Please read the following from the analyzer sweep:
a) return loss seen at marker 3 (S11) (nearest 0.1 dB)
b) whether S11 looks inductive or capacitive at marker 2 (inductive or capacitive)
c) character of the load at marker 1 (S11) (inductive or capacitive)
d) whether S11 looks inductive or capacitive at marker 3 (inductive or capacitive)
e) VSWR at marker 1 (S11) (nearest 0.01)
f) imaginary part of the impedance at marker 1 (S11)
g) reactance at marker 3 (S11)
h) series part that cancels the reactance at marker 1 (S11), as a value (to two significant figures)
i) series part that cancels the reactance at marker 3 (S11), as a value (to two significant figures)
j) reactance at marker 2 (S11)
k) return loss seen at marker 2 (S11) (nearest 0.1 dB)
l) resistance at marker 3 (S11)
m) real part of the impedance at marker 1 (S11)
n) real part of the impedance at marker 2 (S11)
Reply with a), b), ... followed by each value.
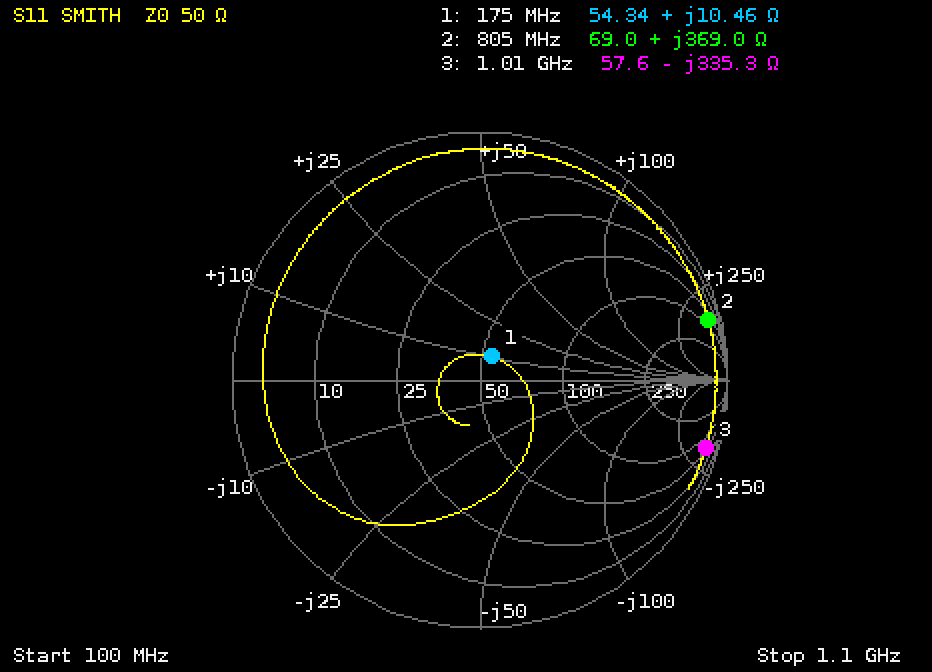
a) 0.4 dB
b) inductive
c) inductive
d) capacitive
e) 1.24
f) +10.46 Ω
g) -335.3 Ω
h) 87 pF
i) 53 nH
j) +369.0 Ω
k) 0.4 dB
l) 57.6 Ω
m) 54.34 Ω
n) 69.0 Ω
